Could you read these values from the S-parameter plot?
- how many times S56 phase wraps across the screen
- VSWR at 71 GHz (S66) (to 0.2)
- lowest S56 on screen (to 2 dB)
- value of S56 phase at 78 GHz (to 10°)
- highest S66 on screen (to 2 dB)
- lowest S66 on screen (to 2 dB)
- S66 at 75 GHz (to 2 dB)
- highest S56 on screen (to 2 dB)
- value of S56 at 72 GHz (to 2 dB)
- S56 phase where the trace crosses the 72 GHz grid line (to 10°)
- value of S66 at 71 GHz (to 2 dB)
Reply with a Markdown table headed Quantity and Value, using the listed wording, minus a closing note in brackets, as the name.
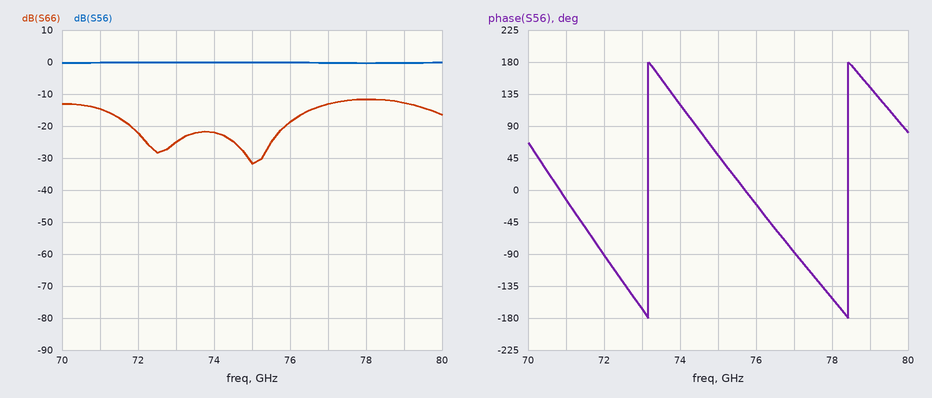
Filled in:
| Quantity | Value |
|---|---|
| how many times S56 phase wraps across the screen | 2 |
| VSWR at 71 GHz (S66) | 1.4 |
| lowest S56 on screen | 0 dB |
| value of S56 phase at 78 GHz | -150° |
| highest S66 on screen | -12 dB |
| lowest S66 on screen | -32 dB |
| S66 at 75 GHz | -32 dB |
| highest S56 on screen | 0 dB |
| value of S56 at 72 GHz | 0 dB |
| S56 phase where the trace crosses the 72 GHz grid line | -90° |
| value of S66 at 71 GHz | -14 dB |
